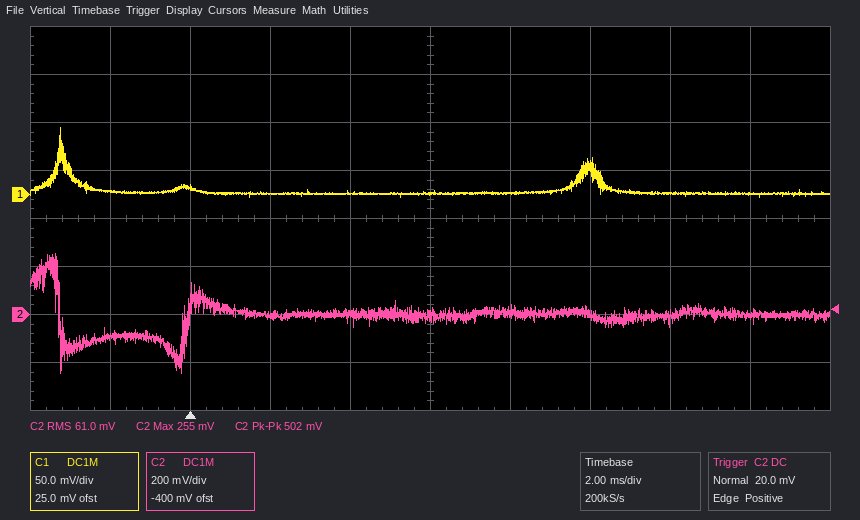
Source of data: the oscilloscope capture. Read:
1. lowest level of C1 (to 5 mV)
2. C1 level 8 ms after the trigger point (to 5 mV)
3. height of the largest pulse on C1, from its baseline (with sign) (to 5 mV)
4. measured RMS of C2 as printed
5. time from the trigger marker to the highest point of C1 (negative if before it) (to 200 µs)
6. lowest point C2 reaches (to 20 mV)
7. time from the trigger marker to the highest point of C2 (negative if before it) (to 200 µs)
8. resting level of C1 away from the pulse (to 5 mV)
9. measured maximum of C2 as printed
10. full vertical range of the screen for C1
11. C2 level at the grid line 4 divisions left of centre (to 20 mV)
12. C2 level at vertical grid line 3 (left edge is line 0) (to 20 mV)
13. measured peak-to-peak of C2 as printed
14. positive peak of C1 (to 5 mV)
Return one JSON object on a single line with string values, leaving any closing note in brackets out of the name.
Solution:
{"lowest level of C1": "-5 mV", "C1 level 8 ms after the trigger point": "0 mV", "height of the largest pulse on C1, from its baseline (with sign)": "+70 mV", "measured RMS of C2 as printed": "61.0 mV", "time from the trigger marker to the highest point of C1 (negative if before it)": "-3.2 ms", "lowest point C2 reaches": "-240 mV", "time from the trigger marker to the highest point of C2 (negative if before it)": "-3.4 ms", "resting level of C1 away from the pulse": "0 mV", "measured maximum of C2 as printed": "255 mV", "full vertical range of the screen for C1": "400 mV", "C2 level at the grid line 4 divisions left of centre": "-100 mV", "C2 level at vertical grid line 3 (left edge is line 0)": "0 mV", "measured peak-to-peak of C2 as printed": "502 mV", "positive peak of C1": "70 mV"}
